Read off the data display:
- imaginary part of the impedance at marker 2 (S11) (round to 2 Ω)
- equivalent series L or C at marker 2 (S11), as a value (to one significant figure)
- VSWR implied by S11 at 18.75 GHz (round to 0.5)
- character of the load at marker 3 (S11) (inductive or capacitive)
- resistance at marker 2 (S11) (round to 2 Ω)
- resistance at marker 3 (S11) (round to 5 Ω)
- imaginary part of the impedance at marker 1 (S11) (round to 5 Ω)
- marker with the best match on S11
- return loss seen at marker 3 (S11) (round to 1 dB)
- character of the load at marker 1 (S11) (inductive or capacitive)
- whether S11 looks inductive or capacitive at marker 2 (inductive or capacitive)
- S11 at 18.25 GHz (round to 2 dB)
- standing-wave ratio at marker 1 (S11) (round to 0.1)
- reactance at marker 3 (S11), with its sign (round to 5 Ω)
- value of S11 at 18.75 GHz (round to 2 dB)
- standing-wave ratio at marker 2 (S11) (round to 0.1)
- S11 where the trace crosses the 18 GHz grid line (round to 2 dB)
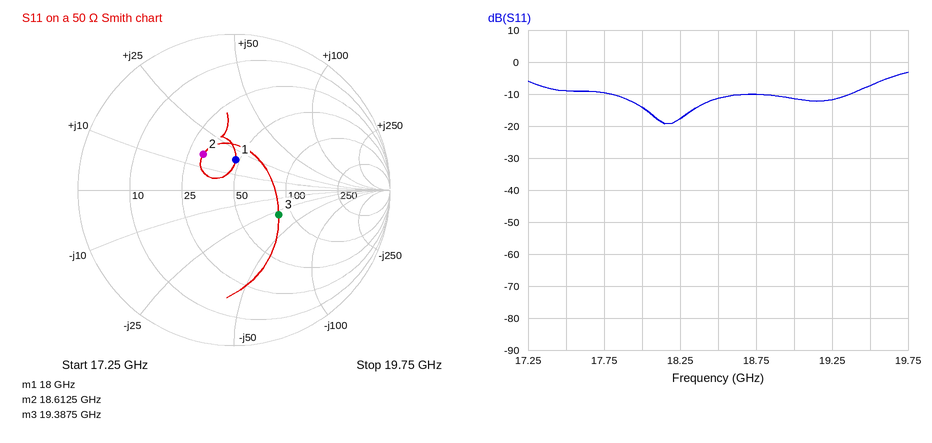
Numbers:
+16 Ω
100 pH
2.0
capacitive
30 Ω
85 Ω
+20 Ω
marker 1
10 dB
inductive
inductive
-18 dB
1.5
-30 Ω
-10 dB
1.9
-14 dB
